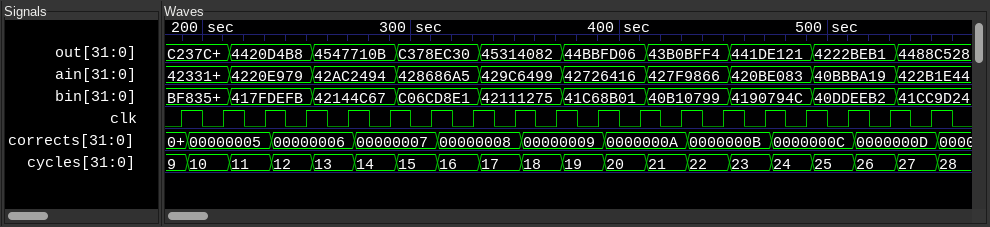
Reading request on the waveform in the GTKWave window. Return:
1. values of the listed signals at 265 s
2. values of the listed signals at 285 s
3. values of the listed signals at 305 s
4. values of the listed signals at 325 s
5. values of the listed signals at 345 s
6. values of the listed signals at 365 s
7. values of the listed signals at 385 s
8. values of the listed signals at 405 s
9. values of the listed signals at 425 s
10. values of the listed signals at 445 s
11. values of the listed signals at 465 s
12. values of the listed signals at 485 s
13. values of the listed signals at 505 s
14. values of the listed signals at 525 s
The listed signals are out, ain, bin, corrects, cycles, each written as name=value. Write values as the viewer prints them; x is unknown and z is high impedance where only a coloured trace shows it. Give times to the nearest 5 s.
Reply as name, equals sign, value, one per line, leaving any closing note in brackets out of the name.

values of the listed signals at 265 s = out=4547710B, ain=42AC2494, bin=42144C67, corrects=00000006, cycles=13
values of the listed signals at 285 s = out=4547710B, ain=42AC2494, bin=42144C67, corrects=00000007, cycles=14
values of the listed signals at 305 s = out=C378EC30, ain=428686A5, bin=C06CD8E1, corrects=00000007, cycles=15
values of the listed signals at 325 s = out=C378EC30, ain=428686A5, bin=C06CD8E1, corrects=00000008, cycles=16
values of the listed signals at 345 s = out=45314082, ain=429C6499, bin=42111275, corrects=00000008, cycles=17
values of the listed signals at 365 s = out=45314082, ain=429C6499, bin=42111275, corrects=00000009, cycles=18
values of the listed signals at 385 s = out=44BBFD06, ain=42726416, bin=41C68B01, corrects=00000009, cycles=19
values of the listed signals at 405 s = out=44BBFD06, ain=42726416, bin=41C68B01, corrects=0000000A, cycles=20
values of the listed signals at 425 s = out=43B0BFF4, ain=427F9866, bin=40B10799, corrects=0000000A, cycles=21
values of the listed signals at 445 s = out=43B0BFF4, ain=427F9866, bin=40B10799, corrects=0000000B, cycles=22
values of the listed signals at 465 s = out=441DE121, ain=420BE083, bin=4190794C, corrects=0000000B, cycles=23
values of the listed signals at 485 s = out=441DE121, ain=420BE083, bin=4190794C, corrects=0000000C, cycles=24
values of the listed signals at 505 s = out=4222BEB1, ain=40BBBA19, bin=40DDEEB2, corrects=0000000C, cycles=25
values of the listed signals at 525 s = out=4222BEB1, ain=40BBBA19, bin=40DDEEB2, corrects=0000000D, cycles=26
